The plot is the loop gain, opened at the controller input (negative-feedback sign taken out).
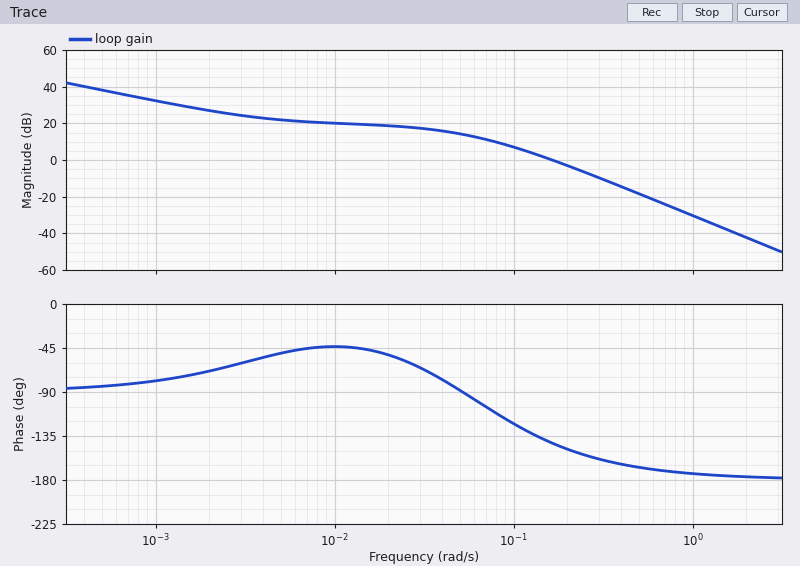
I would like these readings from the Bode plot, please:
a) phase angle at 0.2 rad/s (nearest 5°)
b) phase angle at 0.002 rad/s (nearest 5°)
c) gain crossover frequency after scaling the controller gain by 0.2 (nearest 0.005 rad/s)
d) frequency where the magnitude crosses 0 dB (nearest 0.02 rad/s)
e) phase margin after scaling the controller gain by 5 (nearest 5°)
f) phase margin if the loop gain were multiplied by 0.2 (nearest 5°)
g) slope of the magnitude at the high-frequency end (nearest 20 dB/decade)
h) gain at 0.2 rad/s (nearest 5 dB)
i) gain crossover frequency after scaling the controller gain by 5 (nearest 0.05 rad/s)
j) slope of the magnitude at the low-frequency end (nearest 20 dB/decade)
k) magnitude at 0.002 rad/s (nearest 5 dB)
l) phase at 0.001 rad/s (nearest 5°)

-150°
-70°
0.050 rad/s
0.16 rad/s
15°
90°
-40 dB/decade
-5 dB
0.40 rad/s
-20 dB/decade
25 dB
-80°
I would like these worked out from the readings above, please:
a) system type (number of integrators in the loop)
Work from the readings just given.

1
